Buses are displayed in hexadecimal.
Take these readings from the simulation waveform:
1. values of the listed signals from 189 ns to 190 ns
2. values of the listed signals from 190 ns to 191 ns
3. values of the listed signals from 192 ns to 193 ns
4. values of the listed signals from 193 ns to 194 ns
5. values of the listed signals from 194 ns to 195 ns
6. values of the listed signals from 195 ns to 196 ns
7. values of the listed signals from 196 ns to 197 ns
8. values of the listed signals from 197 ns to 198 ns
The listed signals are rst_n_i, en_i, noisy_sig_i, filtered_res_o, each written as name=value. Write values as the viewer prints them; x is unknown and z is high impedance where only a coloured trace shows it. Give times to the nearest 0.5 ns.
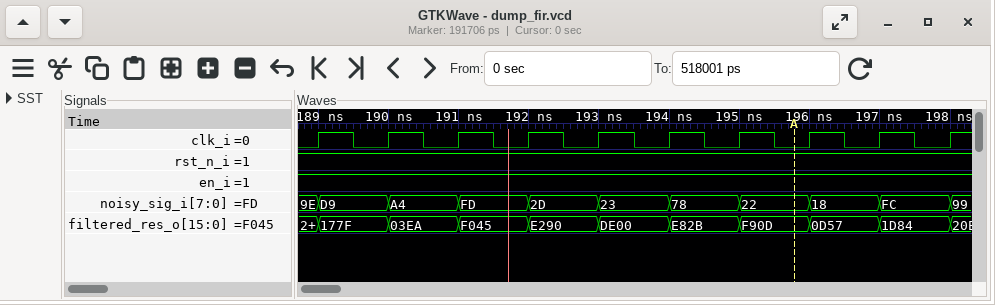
rst_n_i=1, en_i=1, noisy_sig_i=D9, filtered_res_o=177F
rst_n_i=1, en_i=1, noisy_sig_i=A4, filtered_res_o=03EA
rst_n_i=1, en_i=1, noisy_sig_i=2D, filtered_res_o=E290
rst_n_i=1, en_i=1, noisy_sig_i=23, filtered_res_o=DE00
rst_n_i=1, en_i=1, noisy_sig_i=78, filtered_res_o=E82B
rst_n_i=1, en_i=1, noisy_sig_i=22, filtered_res_o=F90D
rst_n_i=1, en_i=1, noisy_sig_i=18, filtered_res_o=0D57
rst_n_i=1, en_i=1, noisy_sig_i=FC, filtered_res_o=1D84
